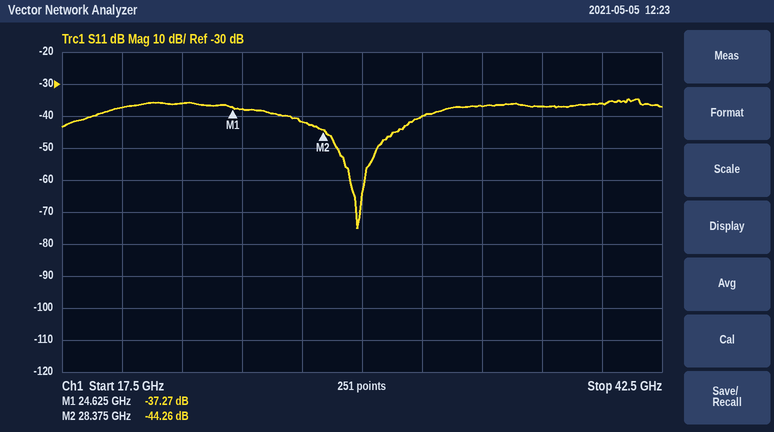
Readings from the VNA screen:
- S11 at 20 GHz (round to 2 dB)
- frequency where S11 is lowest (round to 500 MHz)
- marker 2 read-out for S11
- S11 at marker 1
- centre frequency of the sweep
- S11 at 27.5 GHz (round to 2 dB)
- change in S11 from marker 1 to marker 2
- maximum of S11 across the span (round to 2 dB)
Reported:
-38 dB
30.0 GHz
-44.26 dB
-37.27 dB
30 GHz
-42 dB
-6.99 dB
-34 dB
